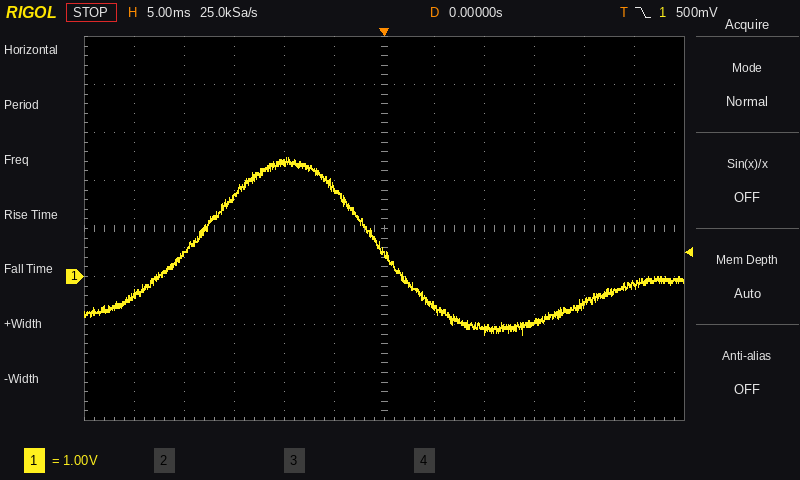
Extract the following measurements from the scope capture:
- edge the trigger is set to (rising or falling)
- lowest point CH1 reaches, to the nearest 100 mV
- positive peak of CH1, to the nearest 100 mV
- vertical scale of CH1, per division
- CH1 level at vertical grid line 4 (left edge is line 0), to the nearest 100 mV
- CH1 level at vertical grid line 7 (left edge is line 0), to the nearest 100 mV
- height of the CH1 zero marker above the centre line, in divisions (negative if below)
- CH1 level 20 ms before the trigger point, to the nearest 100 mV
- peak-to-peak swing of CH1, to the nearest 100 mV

falling
-1.2 V
2.5 V
1 V
2.4 V
-600 mV
-1.0 div
500 mV
3.7 V
